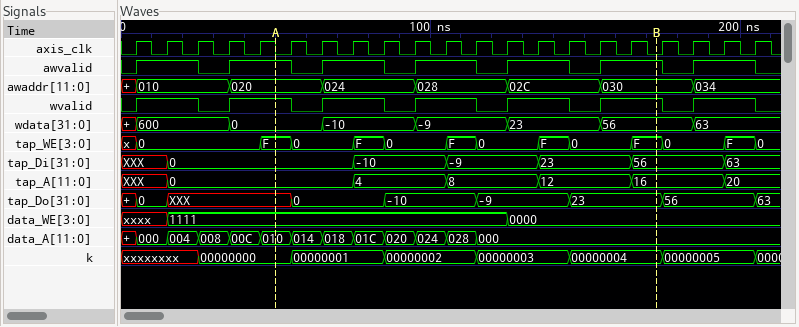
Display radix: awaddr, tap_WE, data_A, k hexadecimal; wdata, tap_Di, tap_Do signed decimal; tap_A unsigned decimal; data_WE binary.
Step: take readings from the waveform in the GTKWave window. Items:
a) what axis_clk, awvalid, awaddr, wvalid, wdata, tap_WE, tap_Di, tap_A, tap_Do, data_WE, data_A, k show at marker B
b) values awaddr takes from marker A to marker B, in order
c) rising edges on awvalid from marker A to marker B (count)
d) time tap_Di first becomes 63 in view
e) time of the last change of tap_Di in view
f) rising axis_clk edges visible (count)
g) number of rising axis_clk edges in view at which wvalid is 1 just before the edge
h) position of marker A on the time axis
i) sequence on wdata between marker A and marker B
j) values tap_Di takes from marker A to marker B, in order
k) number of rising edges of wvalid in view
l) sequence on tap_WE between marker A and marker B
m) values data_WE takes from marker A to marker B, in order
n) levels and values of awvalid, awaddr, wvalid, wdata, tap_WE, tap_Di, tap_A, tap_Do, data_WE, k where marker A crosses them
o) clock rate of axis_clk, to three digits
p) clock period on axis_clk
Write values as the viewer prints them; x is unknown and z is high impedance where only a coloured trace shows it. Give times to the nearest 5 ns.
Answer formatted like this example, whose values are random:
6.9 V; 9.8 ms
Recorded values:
axis_clk=0, awvalid=1, awaddr=030, wvalid=1, wdata=56, tap_WE=F, tap_Di=56, tap_A=16, tap_Do=23, data_WE=0000, data_A=000, k=00000004; 020, 024, 028, 02C, 030; 4; 195 ns; 195 ns; 21; 14; 50 ns; 0, -10, -9, 23, 56; 0, -10, -9, 23, 56; 7; F, 0, F, 0, F, 0, F, 0, F; 1111, 0000; awvalid=1, awaddr=020, wvalid=1, wdata=0, tap_WE=F, tap_Di=0, tap_A=0, tap_Do=XXX, data_WE=1111, k=00000000; 100 MHz; 10 ns
